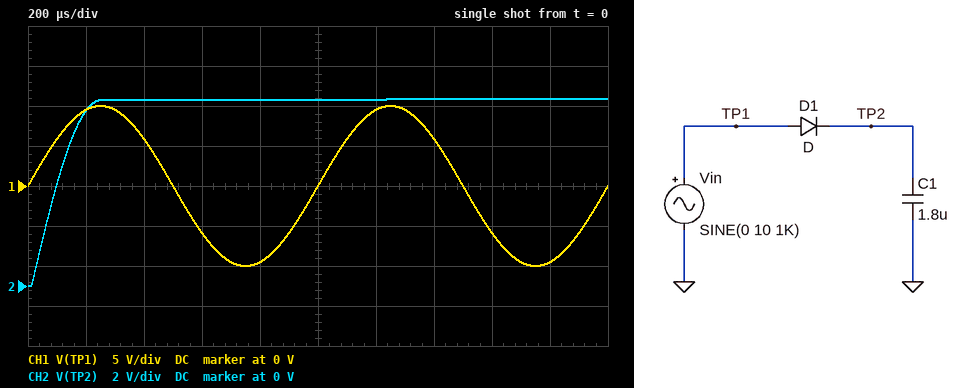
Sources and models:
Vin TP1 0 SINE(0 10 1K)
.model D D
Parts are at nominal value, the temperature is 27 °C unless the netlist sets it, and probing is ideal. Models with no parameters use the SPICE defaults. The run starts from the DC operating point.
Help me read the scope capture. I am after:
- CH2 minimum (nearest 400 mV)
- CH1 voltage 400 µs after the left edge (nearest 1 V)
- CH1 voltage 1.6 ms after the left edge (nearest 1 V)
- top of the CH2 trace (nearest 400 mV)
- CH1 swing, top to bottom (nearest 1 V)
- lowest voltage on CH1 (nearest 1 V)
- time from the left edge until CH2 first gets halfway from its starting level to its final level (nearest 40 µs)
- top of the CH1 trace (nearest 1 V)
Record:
0 V
6 V
-6 V
9.2 V
20 V
-10 V
80 µs
10 V
